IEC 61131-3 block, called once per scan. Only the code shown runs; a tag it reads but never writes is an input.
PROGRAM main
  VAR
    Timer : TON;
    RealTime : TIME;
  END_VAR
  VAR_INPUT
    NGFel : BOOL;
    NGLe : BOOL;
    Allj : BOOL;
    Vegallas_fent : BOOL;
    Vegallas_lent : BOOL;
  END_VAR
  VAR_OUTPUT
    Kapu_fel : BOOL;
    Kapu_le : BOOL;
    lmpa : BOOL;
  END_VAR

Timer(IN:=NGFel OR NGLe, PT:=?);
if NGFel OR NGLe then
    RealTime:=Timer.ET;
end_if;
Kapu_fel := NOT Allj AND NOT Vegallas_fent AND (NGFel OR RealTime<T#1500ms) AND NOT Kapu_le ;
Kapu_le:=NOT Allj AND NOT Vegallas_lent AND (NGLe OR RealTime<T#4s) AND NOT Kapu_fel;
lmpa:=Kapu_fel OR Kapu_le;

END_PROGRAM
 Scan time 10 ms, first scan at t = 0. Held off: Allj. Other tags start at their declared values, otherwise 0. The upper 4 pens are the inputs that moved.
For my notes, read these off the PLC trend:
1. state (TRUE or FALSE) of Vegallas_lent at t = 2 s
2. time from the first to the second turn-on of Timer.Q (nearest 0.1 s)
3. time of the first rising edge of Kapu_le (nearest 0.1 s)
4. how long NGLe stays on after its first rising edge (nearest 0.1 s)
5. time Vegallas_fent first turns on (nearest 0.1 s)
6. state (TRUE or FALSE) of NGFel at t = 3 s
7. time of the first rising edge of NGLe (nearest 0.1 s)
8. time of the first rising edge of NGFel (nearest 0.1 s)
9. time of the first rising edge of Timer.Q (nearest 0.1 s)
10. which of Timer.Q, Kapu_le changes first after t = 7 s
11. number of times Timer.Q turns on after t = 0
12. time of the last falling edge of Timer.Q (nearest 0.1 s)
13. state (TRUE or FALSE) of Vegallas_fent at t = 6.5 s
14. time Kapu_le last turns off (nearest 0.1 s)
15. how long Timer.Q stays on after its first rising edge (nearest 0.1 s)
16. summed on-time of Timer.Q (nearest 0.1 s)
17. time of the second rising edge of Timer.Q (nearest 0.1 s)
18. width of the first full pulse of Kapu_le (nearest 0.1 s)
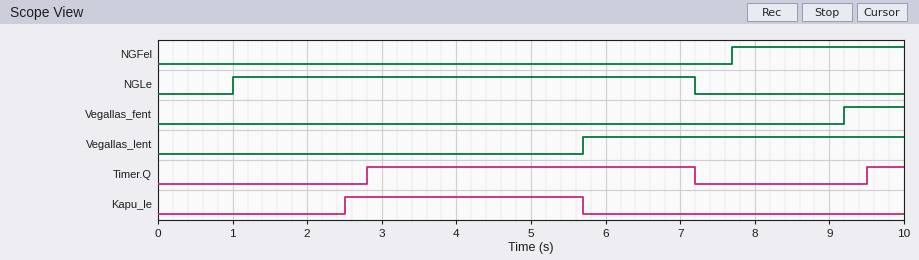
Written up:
FALSE
6.7 s
2.5 s
6.2 s
9.2 s
FALSE
1.0 s
7.7 s
2.8 s
Timer.Q
2
7.2 s
FALSE
5.7 s
4.4 s
4.9 s
9.5 s
3.2 s
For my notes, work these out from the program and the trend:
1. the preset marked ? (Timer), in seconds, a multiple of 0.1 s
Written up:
1.8 s
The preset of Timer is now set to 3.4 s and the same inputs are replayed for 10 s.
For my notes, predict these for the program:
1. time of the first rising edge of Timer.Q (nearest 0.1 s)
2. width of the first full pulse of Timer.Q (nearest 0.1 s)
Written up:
4.4 s
2.8 s
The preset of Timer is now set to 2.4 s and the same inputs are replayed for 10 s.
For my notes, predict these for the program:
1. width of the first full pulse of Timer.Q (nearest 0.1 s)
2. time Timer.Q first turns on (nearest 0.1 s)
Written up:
3.8 s
3.4 s
